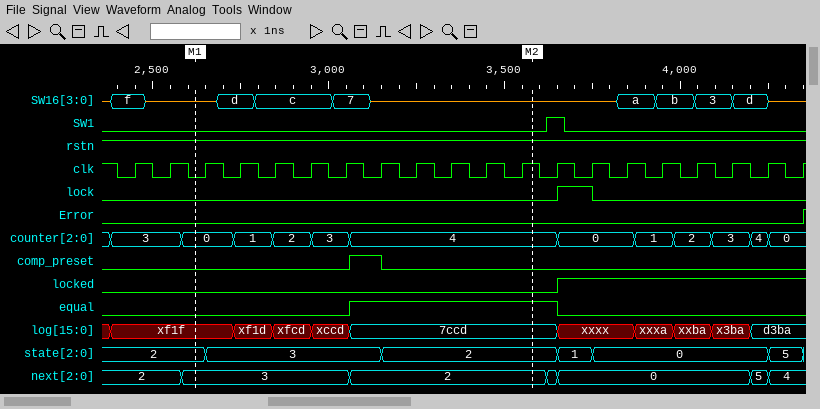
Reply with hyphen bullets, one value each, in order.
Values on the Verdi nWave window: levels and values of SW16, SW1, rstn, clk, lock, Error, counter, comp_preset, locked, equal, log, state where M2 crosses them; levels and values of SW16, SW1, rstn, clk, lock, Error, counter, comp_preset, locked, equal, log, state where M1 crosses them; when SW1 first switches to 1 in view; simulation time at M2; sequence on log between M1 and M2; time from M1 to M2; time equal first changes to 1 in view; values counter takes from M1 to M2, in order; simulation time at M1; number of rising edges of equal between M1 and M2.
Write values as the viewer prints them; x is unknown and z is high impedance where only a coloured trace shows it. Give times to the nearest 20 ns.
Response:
- SW16=z, SW1=0, rstn=1, clk=1, lock=0, Error=0, counter=4, comp_preset=0, locked=0, equal=1, log=7ccd, state=2
- SW16=z, SW1=0, rstn=1, clk=0, lock=0, Error=0, counter=0, comp_preset=0, locked=0, equal=0, log=xf1f, state=2
- 3620 ns
- 3580 ns
- xf1f, xf1d, xfcd, xccd, 7ccd
- 960 ns
- 3060 ns
- 0, 1, 2, 3, 4
- 2620 ns
- 1
